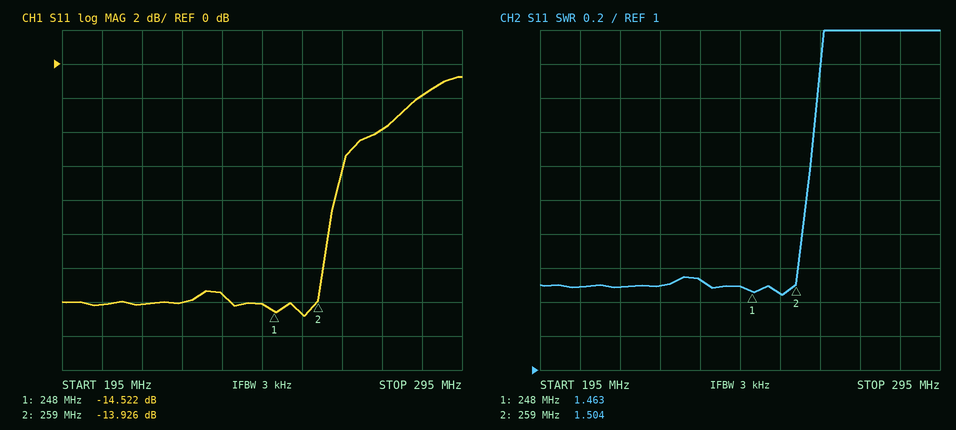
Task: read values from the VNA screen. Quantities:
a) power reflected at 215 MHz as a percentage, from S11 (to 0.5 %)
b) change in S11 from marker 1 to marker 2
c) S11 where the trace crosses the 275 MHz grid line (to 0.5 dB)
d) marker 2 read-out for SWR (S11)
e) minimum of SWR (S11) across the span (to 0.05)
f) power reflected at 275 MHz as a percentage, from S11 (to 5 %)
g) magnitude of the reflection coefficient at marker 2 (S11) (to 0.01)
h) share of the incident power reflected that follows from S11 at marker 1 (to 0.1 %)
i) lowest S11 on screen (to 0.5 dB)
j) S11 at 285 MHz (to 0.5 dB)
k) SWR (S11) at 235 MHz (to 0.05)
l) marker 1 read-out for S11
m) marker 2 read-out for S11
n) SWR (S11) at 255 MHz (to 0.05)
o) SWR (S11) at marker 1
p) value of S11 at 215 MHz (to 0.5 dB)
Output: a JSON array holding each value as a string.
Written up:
["4.0 %", "0.596 dB", "-4.0 dB", "1.504", "1.45", "40 %", "0.20", "3.5 %", "-15.0 dB", "-2.0 dB", "1.55", "-14.522 dB", "-13.926 dB", "1.45", "1.463", "-14.0 dB"]
